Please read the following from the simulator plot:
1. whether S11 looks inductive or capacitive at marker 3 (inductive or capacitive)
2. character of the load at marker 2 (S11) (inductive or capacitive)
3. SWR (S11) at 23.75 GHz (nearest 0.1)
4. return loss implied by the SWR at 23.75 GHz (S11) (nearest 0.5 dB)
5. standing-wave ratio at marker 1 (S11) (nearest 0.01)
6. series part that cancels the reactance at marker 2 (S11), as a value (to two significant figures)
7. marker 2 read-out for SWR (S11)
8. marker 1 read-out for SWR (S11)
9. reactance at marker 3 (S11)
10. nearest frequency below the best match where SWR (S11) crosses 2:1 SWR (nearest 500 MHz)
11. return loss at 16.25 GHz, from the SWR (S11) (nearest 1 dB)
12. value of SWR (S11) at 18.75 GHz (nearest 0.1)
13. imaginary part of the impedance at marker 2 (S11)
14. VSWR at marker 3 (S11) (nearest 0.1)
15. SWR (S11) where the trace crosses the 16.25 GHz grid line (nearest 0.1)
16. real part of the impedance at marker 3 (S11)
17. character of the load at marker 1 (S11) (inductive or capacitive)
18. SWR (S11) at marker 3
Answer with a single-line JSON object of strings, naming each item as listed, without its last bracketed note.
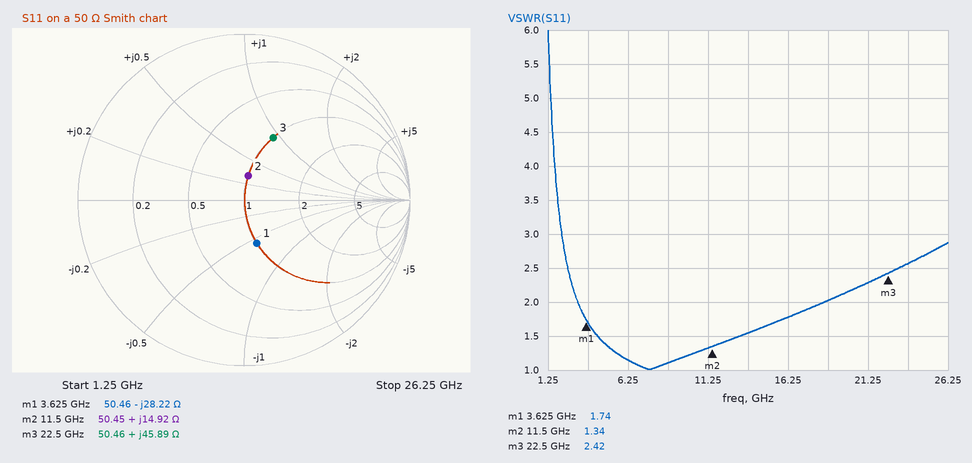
{"whether S11 looks inductive or capacitive at marker 3": "inductive", "character of the load at marker 2 (S11)": "inductive", "SWR (S11) at 23.75 GHz": "2.6", "return loss implied by the SWR at 23.75 GHz (S11)": "7.0 dB", "standing-wave ratio at marker 1 (S11)": "1.74", "series part that cancels the reactance at marker 2 (S11), as a value": "930 fF", "marker 2 read-out for SWR": "1.34", "marker 1 read-out for SWR": "1.74", "reactance at marker 3": "+45.89 Ω", "nearest frequency below the best match where SWR (S11) crosses 2:1 SWR": "3.0 GHz", "return loss at 16.25 GHz, from the SWR (S11)": "11 dB", "value of SWR (S11) at 18.75 GHz": "2.0", "imaginary part of the impedance at marker 2": "+14.92 Ω", "VSWR at marker 3 (S11)": "2.4", "SWR (S11) where the trace crosses the 16.25 GHz grid line": "1.8", "real part of the impedance at marker 3": "50.46 Ω", "character of the load at marker 1 (S11)": "capacitive", "SWR (S11) at marker 3": "2.42"}
